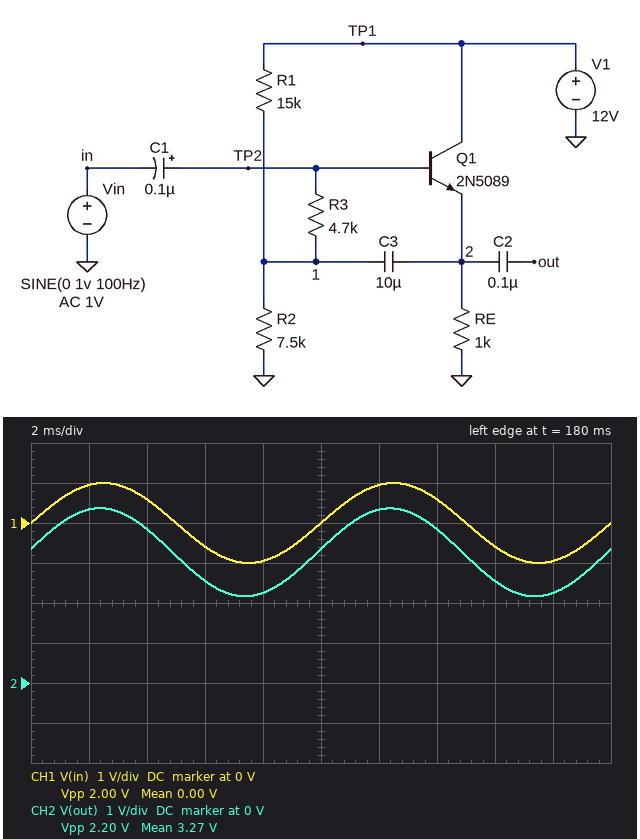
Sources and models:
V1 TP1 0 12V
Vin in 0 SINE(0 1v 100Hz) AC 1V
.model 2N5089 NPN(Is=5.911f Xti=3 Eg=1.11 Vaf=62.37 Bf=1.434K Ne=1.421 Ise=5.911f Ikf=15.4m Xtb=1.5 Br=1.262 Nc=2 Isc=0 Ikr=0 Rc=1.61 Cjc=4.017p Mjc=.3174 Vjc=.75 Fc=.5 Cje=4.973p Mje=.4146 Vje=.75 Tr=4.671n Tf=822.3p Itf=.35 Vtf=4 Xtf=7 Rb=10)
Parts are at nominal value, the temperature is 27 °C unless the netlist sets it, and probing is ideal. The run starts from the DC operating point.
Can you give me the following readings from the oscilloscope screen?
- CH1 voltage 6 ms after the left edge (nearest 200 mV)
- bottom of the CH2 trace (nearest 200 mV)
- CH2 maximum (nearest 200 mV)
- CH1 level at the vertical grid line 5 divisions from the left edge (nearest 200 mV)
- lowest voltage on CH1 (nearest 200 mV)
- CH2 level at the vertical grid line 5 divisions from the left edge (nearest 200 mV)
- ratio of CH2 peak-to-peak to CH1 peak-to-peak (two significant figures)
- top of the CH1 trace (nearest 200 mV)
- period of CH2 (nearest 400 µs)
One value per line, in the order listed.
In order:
-600 mV
2.2 V
4.4 V
0 V
-1.0 V
3.4 V
1.1
1.0 V
10.0 ms
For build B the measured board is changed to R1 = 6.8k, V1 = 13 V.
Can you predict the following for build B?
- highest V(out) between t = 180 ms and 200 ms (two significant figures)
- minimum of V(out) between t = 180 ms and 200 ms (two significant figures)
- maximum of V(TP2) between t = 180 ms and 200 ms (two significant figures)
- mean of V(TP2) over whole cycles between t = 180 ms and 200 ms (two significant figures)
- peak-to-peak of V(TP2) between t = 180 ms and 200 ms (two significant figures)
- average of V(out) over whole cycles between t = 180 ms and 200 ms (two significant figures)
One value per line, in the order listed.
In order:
7.2 V
4.9 V
7.9 V
6.8 V
2.3 V
6.0 V
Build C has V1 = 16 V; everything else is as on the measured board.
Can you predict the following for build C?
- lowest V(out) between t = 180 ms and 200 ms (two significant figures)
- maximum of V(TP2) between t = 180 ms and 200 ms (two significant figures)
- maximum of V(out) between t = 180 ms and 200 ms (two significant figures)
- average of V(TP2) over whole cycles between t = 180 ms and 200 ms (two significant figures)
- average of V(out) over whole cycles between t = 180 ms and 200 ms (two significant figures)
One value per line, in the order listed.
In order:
3.5 V
6.4 V
5.7 V
5.3 V
4.6 V
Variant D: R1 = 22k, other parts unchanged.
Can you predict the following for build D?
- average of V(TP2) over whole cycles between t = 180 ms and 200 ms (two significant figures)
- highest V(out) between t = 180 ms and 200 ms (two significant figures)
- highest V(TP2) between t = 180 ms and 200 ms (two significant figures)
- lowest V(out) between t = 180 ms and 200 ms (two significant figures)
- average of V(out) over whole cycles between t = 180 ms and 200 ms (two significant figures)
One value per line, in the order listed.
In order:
3.0 V
3.4 V
4.1 V
1.3 V
2.3 V
